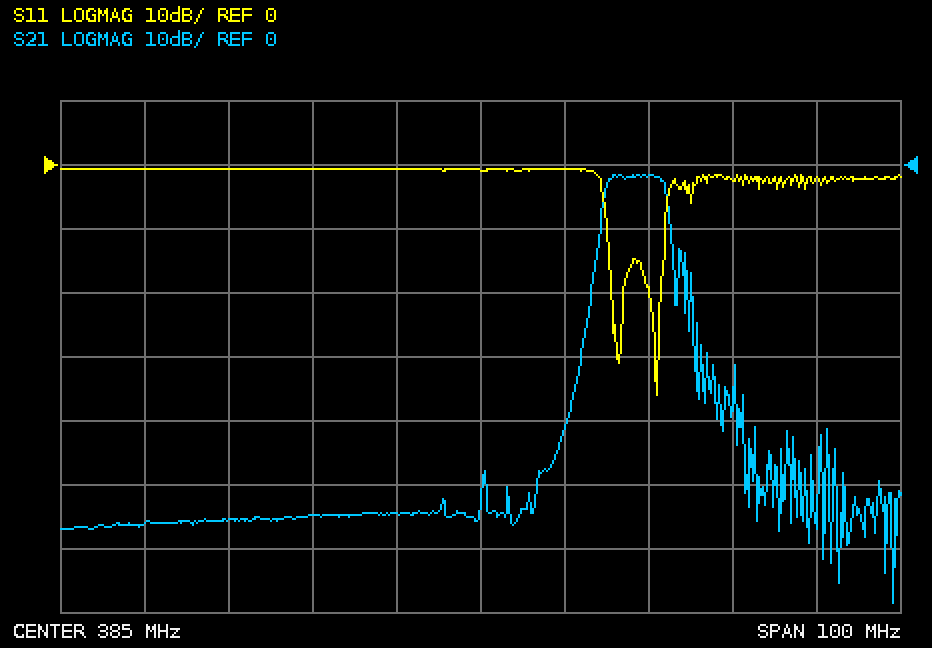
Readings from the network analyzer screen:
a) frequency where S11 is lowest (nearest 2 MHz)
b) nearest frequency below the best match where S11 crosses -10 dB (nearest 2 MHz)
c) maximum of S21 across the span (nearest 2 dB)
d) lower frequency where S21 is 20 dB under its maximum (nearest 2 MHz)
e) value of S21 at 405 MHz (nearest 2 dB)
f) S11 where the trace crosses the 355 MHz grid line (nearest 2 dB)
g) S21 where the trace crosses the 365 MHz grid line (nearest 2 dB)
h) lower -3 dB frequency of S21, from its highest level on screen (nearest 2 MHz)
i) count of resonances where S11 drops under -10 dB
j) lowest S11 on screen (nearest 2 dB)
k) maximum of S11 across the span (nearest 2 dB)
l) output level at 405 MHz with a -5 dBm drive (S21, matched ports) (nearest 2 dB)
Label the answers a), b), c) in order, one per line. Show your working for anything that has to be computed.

a) 406 MHz
b) 400 MHz
c) -2 dB
d) 398 MHz
e) -2 dB
f) 0 dB
g) -54 dB
h) 400 MHz
i) 2
j) -36 dB
k) 0 dB
l) -5 dBm + (-2 dB) = -6 dBm
